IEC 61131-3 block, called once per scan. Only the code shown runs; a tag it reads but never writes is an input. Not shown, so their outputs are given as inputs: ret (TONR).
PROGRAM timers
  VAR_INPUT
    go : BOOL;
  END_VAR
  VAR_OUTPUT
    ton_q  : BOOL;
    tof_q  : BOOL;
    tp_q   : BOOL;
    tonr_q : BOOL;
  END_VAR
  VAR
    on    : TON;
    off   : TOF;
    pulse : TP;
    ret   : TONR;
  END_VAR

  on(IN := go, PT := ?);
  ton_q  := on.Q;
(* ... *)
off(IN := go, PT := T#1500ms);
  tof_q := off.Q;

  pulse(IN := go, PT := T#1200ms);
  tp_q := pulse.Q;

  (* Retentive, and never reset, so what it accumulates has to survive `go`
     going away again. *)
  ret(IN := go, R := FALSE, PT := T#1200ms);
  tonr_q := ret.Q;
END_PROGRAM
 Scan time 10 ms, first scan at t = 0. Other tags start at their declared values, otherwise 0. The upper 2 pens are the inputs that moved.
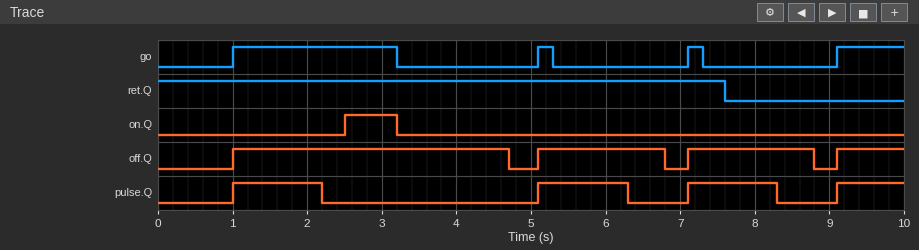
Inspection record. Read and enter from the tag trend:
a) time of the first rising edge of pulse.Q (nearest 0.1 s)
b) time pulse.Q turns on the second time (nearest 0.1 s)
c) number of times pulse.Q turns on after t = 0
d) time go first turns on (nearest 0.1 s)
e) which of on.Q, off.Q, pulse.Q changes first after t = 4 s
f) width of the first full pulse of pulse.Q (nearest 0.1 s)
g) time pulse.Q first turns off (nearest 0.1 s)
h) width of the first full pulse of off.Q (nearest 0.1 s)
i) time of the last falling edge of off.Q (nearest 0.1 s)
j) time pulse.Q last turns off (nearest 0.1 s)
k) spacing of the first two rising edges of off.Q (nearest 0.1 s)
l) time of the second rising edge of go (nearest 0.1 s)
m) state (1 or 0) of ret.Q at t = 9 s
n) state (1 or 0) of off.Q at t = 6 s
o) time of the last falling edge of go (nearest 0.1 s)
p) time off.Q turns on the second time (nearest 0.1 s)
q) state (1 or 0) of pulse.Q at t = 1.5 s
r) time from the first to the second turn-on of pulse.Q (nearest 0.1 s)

1.0 s
5.1 s
4
1.0 s
off.Q
1.2 s
2.2 s
3.7 s
8.8 s
8.3 s
4.1 s
5.1 s
0
1
7.3 s
5.1 s
1
4.1 s
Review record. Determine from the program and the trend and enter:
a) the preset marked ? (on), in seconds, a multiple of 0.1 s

1.5 s
